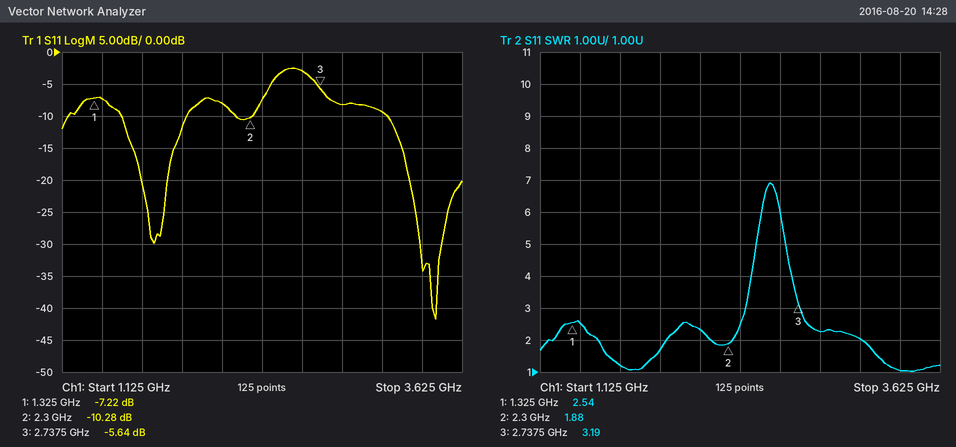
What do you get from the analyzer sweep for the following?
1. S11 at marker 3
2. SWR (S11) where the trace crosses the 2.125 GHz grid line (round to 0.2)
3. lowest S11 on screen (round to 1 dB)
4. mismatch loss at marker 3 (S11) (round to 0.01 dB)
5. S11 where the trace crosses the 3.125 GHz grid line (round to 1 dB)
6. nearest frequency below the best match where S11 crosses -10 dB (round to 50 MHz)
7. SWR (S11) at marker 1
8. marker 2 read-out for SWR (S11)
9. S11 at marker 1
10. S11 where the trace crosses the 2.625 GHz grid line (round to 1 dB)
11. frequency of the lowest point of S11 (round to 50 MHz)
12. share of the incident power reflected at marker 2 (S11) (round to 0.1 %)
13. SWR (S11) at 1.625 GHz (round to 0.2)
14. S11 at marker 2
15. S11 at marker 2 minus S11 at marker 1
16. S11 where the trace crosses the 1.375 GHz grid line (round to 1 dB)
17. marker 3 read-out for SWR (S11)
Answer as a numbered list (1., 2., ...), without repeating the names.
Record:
1. -5.64 dB
2. 2.4
3. -42 dB
4. 1.38 dB
5. -9 dB
6. 3.15 GHz
7. 2.54
8. 1.88
9. -7.22 dB
10. -3 dB
11. 3.45 GHz
12. 9.4 %
13. 1.2
14. -10.28 dB
15. -3.06 dB
16. -7 dB
17. 3.19
